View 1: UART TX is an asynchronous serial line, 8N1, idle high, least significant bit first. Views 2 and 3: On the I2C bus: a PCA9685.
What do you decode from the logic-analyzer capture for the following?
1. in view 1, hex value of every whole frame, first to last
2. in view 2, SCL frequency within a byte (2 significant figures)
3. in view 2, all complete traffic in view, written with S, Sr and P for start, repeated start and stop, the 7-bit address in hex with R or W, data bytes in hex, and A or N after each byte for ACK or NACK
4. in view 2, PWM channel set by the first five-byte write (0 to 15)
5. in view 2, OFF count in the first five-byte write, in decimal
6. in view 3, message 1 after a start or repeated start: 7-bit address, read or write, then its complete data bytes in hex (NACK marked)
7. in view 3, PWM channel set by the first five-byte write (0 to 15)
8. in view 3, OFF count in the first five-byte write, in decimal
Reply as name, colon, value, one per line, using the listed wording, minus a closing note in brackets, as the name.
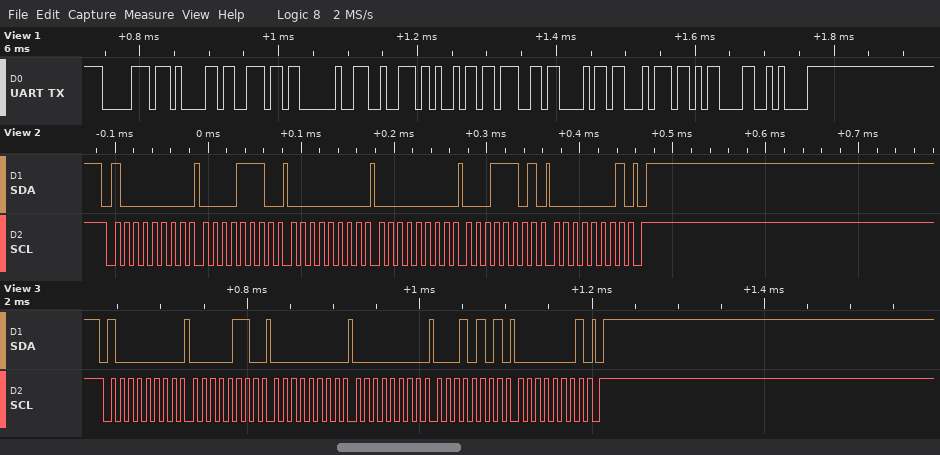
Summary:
in view 1, hex value of every whole frame, first to last: 70 61 6E 20 72 69 67 68 74 0D 0A
in view 2, SCL frequency within a byte: 100 kHz
in view 2, all complete traffic in view, written with S, Sr and P for start, repeated start and stop, the 7-bit address in hex with R or W, data bytes in hex, and A or N after each byte for ACK or NACK: S 40W A 0E A 00 A 00 A 1D A 01 A P
in view 2, PWM channel set by the first five-byte write: 2
in view 2, OFF count in the first five-byte write, in decimal: 285
in view 3, message 1 after a start or repeated start: 7-bit address, read or write, then its complete data bytes in hex: 0x40 write: 06 00 00 15 01
in view 3, PWM channel set by the first five-byte write: 0
in view 3, OFF count in the first five-byte write, in decimal: 277
